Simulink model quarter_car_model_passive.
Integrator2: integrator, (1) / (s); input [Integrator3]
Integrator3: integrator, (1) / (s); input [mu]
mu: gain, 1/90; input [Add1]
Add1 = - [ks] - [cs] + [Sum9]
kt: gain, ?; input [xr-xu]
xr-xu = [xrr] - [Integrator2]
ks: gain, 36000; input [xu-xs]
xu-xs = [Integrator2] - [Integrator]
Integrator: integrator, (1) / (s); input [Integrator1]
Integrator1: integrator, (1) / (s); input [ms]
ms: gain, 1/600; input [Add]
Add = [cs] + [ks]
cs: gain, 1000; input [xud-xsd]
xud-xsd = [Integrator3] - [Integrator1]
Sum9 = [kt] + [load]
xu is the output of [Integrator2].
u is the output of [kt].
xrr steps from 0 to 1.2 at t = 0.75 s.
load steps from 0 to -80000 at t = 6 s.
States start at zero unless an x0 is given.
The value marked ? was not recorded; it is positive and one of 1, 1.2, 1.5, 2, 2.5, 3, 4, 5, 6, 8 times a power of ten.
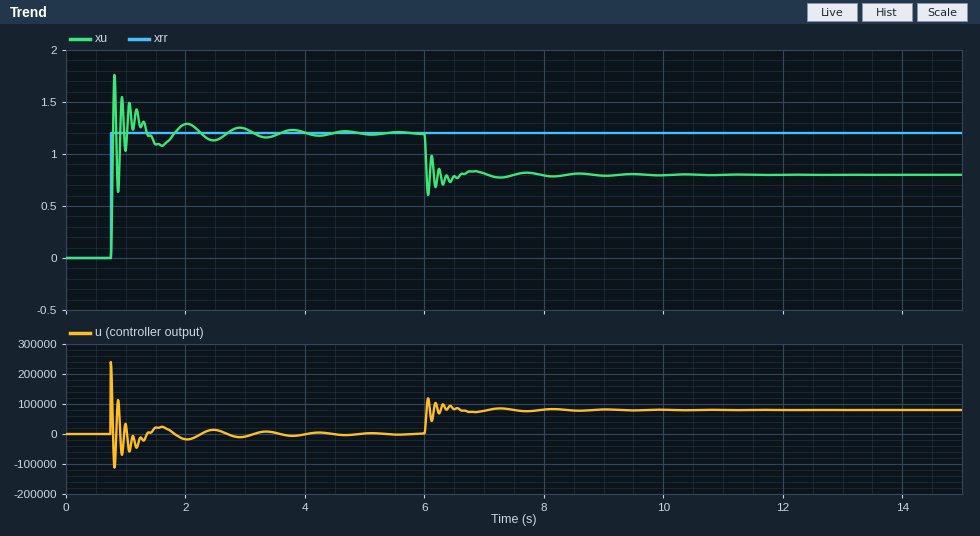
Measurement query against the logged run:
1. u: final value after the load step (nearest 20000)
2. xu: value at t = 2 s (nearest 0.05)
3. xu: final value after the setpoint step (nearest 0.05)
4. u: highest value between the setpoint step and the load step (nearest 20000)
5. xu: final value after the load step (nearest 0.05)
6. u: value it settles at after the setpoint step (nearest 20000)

80000
1.30
1.20
240000
0.80
0
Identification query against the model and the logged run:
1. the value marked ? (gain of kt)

200000
